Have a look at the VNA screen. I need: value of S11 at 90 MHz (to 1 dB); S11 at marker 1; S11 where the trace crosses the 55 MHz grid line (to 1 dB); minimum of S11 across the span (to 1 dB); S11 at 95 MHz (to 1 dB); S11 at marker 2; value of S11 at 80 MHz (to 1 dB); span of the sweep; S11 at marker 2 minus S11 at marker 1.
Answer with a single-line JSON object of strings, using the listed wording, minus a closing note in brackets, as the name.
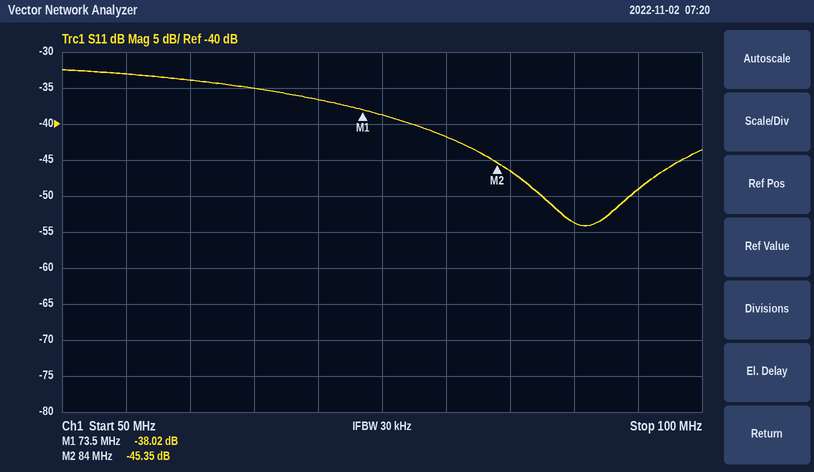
{"value of S11 at 90 MHz": "-54 dB", "S11 at marker 1": "-38.02 dB", "S11 where the trace crosses the 55 MHz grid line": "-33 dB", "minimum of S11 across the span": "-54 dB", "S11 at 95 MHz": "-49 dB", "S11 at marker 2": "-45.35 dB", "value of S11 at 80 MHz": "-42 dB", "span of the sweep": "50 MHz", "S11 at marker 2 minus S11 at marker 1": "-7.33 dB"}
